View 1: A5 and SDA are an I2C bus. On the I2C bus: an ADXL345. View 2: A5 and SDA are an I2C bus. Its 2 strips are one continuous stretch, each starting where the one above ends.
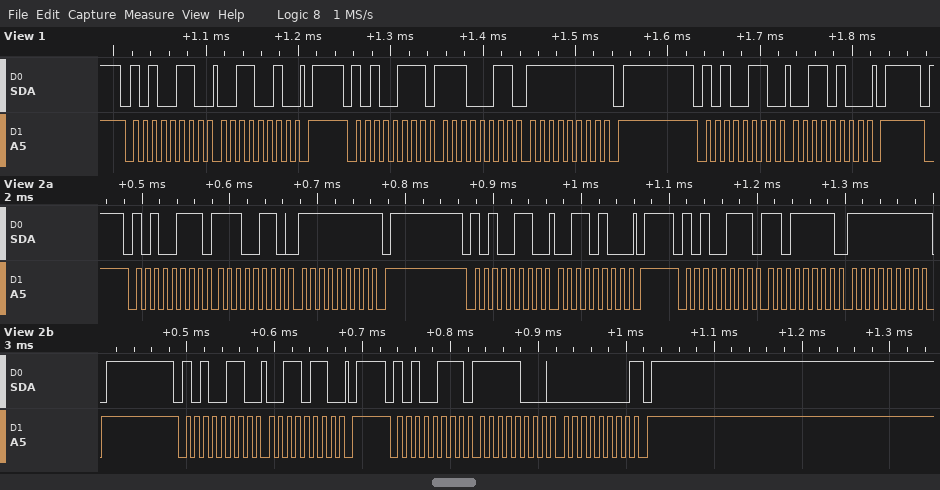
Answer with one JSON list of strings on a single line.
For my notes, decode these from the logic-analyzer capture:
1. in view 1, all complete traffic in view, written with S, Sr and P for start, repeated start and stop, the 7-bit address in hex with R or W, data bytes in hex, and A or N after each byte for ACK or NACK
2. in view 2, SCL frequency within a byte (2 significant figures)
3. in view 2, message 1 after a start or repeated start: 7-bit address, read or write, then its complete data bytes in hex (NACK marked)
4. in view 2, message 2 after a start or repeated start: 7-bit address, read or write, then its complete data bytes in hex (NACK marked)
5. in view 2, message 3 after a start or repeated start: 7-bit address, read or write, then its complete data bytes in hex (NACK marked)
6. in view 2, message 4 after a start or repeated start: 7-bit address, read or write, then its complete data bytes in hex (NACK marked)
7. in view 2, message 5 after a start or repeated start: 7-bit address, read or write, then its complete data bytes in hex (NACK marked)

["S 53W A 32 A P S 53R A E3 A FF N P S 53W A 34 A P", "100 kHz", "0x53 read: E6 FF NACK", "0x53 write: 34", "0x53 read: DF FF NACK", "0x53 write: 36", "0x53 read: F8 00 NACK"]
